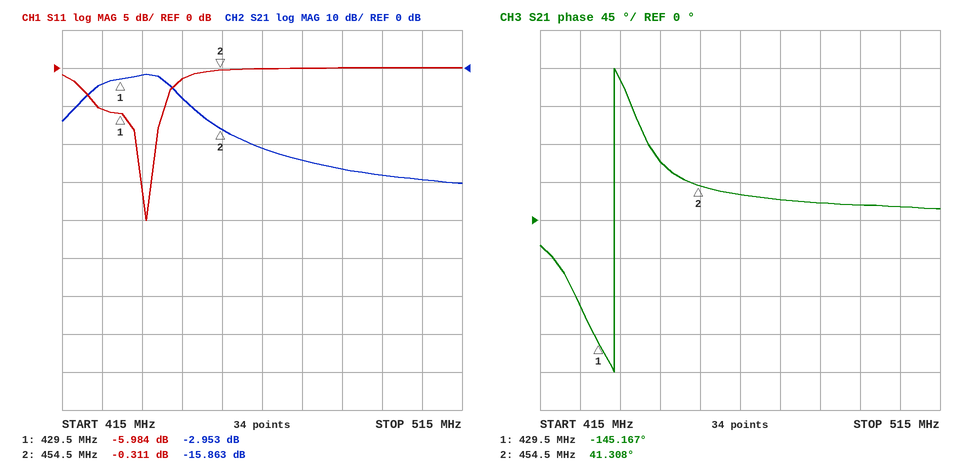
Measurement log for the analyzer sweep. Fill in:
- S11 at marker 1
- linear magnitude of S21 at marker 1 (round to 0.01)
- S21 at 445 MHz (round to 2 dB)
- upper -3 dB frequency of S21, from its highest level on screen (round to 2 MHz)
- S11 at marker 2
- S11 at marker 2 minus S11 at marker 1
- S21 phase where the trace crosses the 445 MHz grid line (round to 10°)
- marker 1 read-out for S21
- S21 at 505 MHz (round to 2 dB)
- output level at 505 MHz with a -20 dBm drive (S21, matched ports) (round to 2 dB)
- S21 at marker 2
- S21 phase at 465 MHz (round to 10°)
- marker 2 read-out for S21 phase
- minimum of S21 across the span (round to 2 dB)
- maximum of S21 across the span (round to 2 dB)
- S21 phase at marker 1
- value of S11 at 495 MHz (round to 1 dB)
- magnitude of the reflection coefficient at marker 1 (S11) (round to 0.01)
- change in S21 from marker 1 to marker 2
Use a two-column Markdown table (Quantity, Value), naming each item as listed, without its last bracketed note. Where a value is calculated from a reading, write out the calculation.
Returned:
| Quantity | Value |
|---|---|
| S11 at marker 1 | -5.984 dB |
| linear magnitude of S21 at marker 1 | 10^(-2.953/20) ≈ 0.71 |
| S21 at 445 MHz | -8 dB |
| upper -3 dB frequency of S21, from its highest level on screen | 442 MHz |
| S11 at marker 2 | -0.311 dB |
| S11 at marker 2 minus S11 at marker 1 | -0.311 − (-5.984) = 5.673 dB |
| S21 phase where the trace crosses the 445 MHz grid line | 70° |
| marker 1 read-out for S21 | -2.953 dB |
| S21 at 505 MHz | -30 dB |
| output level at 505 MHz with a -20 dBm drive (S21, matched ports) | -20 dBm + (-30 dB) = -50 dBm |
| S21 at marker 2 | -15.863 dB |
| S21 phase at 465 MHz | 30° |
| marker 2 read-out for S21 phase | 41.308° |
| minimum of S21 across the span | -30 dB |
| maximum of S21 across the span | -2 dB |
| S21 phase at marker 1 | -145.167° |
| value of S11 at 495 MHz | 0 dB |
| magnitude of the reflection coefficient at marker 1 (S11) | 10^(-5.984/20) ≈ 0.50 |
| change in S21 from marker 1 to marker 2 | -15.863 − (-2.953) = -12.910 dB |
